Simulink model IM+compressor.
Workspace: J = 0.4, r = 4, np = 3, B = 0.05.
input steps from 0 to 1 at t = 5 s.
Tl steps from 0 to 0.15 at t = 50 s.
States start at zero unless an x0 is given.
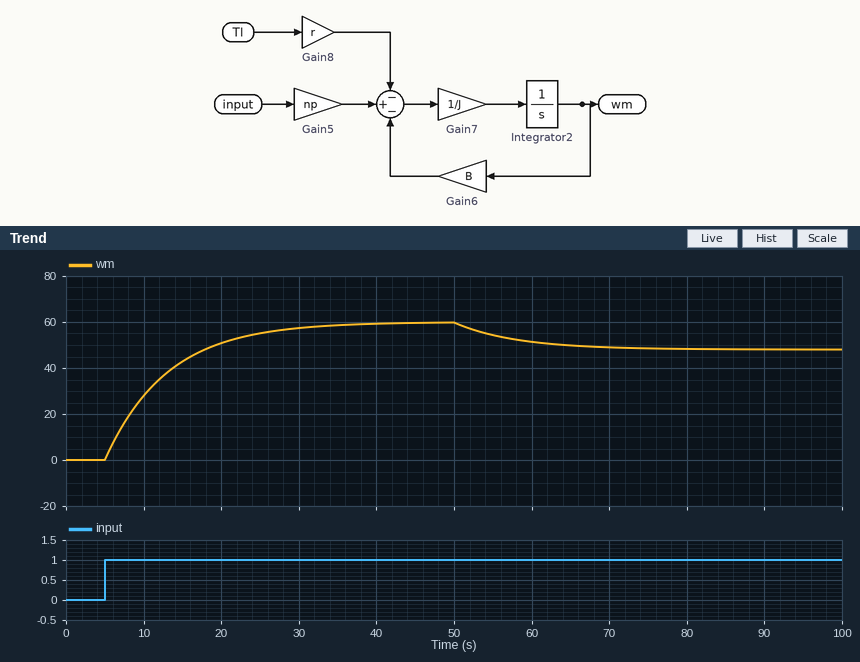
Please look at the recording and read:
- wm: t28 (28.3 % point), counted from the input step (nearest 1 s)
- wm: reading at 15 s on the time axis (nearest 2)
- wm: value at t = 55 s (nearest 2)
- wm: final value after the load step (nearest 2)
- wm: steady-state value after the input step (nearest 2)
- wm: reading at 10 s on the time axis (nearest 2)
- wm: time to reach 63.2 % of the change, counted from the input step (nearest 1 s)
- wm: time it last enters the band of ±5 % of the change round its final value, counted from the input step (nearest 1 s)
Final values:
3 s
42
54
48
60
28
8 s
24 s
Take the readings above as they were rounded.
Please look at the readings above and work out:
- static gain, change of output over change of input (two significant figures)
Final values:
60
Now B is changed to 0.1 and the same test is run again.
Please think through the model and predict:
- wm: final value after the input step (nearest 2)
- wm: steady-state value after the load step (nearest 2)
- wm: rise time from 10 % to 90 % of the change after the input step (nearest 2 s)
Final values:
30
24
8 s
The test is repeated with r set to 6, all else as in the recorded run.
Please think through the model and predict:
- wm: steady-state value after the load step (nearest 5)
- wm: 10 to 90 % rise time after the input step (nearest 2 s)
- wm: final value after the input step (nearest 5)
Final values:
40
18 s
60
